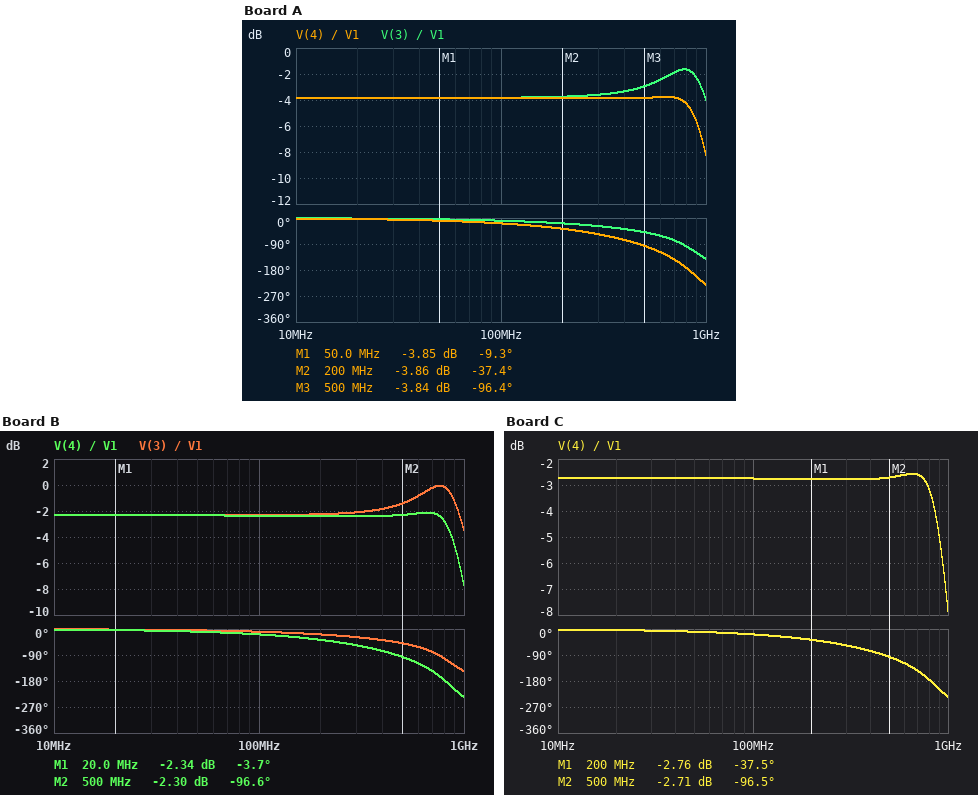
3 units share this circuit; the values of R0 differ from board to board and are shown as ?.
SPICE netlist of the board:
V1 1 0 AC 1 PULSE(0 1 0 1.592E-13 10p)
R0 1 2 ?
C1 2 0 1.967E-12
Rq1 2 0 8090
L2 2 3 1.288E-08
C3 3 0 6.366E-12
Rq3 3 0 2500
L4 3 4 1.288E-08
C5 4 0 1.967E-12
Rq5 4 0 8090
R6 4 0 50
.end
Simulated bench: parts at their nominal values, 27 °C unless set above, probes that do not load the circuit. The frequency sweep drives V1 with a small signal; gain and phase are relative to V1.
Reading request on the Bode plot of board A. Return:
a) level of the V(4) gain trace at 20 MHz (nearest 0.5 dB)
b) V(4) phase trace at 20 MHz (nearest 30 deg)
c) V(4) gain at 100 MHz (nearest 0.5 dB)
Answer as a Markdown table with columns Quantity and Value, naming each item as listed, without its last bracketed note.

| Quantity | Value |
|---|---|
| level of the V(4) gain trace at 20 MHz | -4.0 dB |
| V(4) phase trace at 20 MHz | 0 deg |
| V(4) gain at 100 MHz | -4.0 dB |
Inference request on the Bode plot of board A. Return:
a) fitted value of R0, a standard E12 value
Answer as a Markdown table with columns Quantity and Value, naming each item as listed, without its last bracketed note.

| Quantity | Value |
|---|---|
| fitted value of R0, a standard E12 value | 27 Ω |
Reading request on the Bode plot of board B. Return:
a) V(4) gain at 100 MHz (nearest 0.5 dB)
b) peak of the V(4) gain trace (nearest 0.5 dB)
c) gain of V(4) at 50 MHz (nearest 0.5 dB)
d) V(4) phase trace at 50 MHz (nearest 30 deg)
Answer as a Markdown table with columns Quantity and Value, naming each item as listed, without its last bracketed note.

| Quantity | Value |
|---|---|
| V(4) gain at 100 MHz | -2.5 dB |
| peak of the V(4) gain trace | -2.0 dB |
| gain of V(4) at 50 MHz | -2.5 dB |
| V(4) phase trace at 50 MHz | 0 deg |
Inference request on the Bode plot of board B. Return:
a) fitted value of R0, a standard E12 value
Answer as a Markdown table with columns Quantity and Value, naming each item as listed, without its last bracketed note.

| Quantity | Value |
|---|---|
| fitted value of R0, a standard E12 value | 15 Ω |
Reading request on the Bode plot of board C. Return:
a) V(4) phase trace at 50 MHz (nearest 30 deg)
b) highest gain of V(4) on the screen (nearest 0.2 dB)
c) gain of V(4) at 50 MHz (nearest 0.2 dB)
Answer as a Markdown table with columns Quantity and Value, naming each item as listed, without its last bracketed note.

| Quantity | Value |
|---|---|
| V(4) phase trace at 50 MHz | 0 deg |
| highest gain of V(4) on the screen | -2.6 dB |
| gain of V(4) at 50 MHz | -2.8 dB |
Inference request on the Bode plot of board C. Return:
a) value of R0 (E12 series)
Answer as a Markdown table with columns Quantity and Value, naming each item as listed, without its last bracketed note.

| Quantity | Value |
|---|---|
| value of R0 | 18 Ω |
